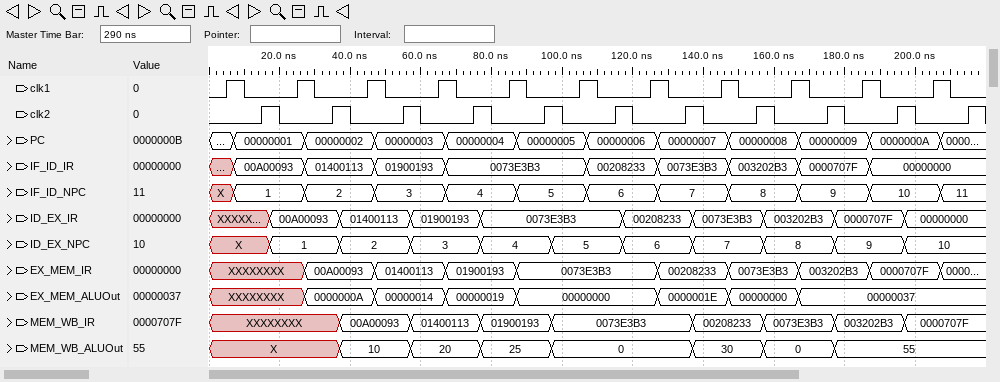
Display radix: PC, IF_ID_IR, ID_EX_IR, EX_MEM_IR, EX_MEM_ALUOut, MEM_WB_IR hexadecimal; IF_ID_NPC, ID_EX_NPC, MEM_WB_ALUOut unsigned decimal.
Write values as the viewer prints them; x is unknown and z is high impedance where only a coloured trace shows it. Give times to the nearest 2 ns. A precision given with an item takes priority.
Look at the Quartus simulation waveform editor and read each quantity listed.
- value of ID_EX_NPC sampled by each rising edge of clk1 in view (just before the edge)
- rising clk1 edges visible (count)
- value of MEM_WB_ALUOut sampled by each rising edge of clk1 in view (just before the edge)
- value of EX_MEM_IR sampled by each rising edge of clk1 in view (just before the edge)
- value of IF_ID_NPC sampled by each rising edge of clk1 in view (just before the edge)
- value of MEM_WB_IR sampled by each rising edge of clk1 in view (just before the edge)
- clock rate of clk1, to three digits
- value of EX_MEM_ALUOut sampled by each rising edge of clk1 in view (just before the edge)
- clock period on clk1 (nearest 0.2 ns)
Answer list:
X, 1, 2, 3, 4, 5, 6, 7, 8, 9, 10
11
X, X, 10, 20, 25, 0, 0, 30, 0, 55, 55
XXXXXXXX, XXXXXXXX, 00A00093, 01400113, 01900193, 0073E3B3, 0073E3B3, 00208233, 0073E3B3, 003202B3, 0000707F
X, 1, 2, 3, 4, 5, 6, 7, 8, 9, 10
XXXXXXXX, XXXXXXXX, 00A00093, 01400113, 01900193, 0073E3B3, 0073E3B3, 00208233, 0073E3B3, 003202B3, 0000707F
50.0 MHz
XXXXXXXX, XXXXXXXX, 0000000A, 00000014, 00000019, 00000000, 00000000, 0000001E, 00000000, 00000037, 00000037
20 ns
